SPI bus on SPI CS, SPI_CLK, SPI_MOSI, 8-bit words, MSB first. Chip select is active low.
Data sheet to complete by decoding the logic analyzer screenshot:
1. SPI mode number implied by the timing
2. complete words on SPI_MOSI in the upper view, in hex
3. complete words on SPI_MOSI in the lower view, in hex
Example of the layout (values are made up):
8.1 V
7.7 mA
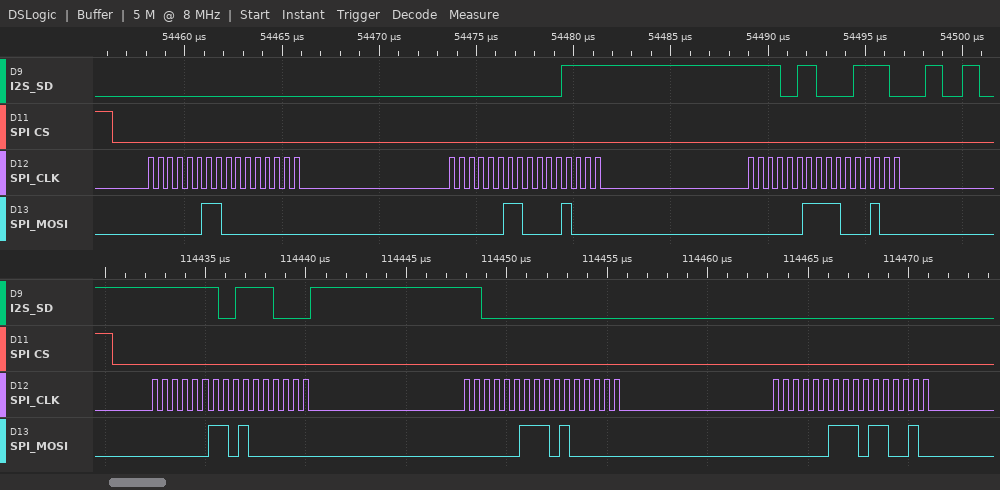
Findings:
0
03, 00, 03, 08, 03, C4
03, 40, 03, A0, 03, B2
